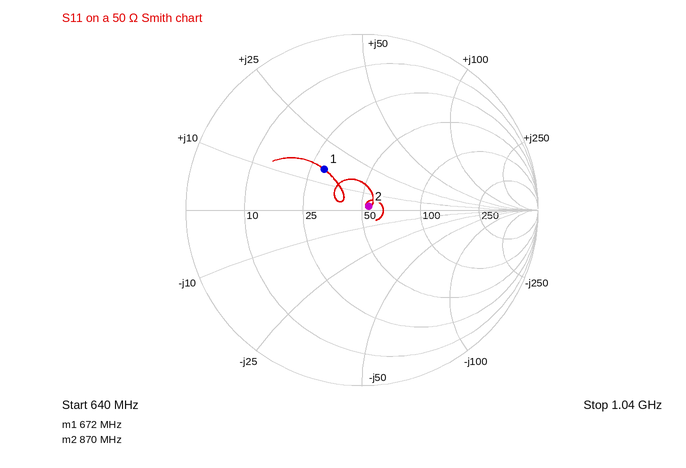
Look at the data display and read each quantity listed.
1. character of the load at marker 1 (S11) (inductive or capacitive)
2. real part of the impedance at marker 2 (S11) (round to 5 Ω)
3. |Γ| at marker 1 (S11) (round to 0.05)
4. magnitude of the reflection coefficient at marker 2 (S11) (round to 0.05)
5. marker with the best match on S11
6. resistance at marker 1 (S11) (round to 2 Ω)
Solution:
inductive
55 Ω
0.30
0.05
marker 2
30 Ω
